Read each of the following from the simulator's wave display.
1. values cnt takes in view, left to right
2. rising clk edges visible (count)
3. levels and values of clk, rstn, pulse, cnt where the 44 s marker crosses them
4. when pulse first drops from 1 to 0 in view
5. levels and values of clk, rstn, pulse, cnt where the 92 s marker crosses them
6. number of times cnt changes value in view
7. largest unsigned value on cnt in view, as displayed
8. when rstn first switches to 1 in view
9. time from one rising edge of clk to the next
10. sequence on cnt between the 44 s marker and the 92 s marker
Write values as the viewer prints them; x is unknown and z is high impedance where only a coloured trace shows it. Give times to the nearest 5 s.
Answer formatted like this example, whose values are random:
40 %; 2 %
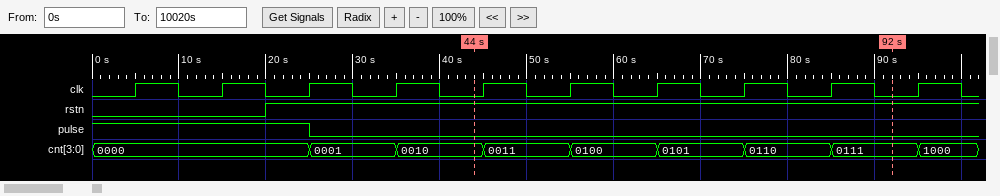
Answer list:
0000, 0001, 0010, 0011, 0100, 0101, 0110, 0111, 1000; 10; clk=0, rstn=1, pulse=0, cnt=0010; 25 s; clk=0, rstn=1, pulse=0, cnt=0111; 8; 1000; 20 s; 10 s; 0010, 0011, 0100, 0101, 0110, 0111
